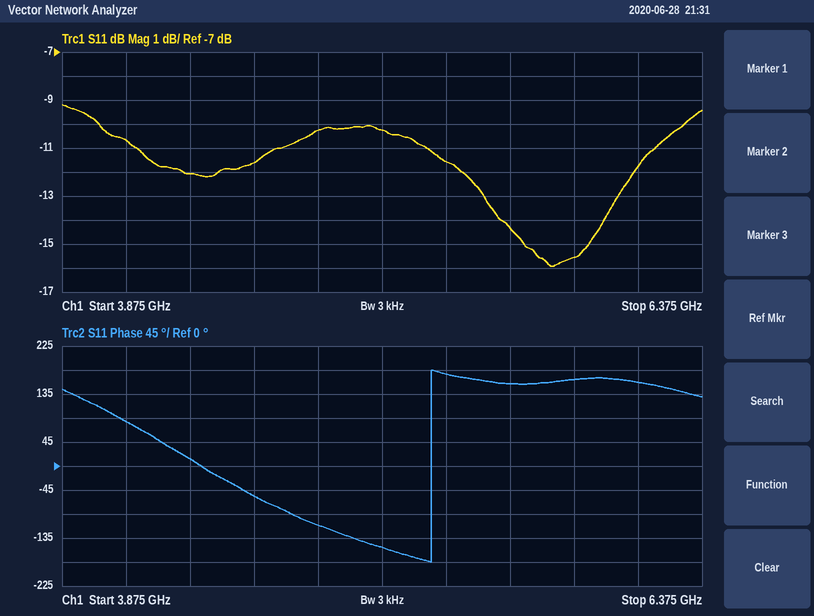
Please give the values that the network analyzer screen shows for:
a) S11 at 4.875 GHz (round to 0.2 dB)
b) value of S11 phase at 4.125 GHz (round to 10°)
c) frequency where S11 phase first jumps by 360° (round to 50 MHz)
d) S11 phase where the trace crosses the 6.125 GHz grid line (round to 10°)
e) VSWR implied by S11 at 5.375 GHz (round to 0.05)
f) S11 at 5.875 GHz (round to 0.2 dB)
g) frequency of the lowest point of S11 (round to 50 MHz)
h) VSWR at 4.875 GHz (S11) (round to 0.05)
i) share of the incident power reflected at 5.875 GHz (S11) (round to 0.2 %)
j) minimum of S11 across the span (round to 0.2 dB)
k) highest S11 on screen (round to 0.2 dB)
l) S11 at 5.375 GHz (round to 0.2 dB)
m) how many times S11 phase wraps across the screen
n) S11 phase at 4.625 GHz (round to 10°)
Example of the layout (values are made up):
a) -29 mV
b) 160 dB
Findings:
a) -10.2 dB
b) 80°
c) 5.30 GHz
d) 160°
e) 1.70
f) -15.6 dB
g) 5.80 GHz
h) 1.90
i) 2.8 %
j) -16.0 dB
k) -9.2 dB
l) -11.6 dB
m) 1
n) -60°
